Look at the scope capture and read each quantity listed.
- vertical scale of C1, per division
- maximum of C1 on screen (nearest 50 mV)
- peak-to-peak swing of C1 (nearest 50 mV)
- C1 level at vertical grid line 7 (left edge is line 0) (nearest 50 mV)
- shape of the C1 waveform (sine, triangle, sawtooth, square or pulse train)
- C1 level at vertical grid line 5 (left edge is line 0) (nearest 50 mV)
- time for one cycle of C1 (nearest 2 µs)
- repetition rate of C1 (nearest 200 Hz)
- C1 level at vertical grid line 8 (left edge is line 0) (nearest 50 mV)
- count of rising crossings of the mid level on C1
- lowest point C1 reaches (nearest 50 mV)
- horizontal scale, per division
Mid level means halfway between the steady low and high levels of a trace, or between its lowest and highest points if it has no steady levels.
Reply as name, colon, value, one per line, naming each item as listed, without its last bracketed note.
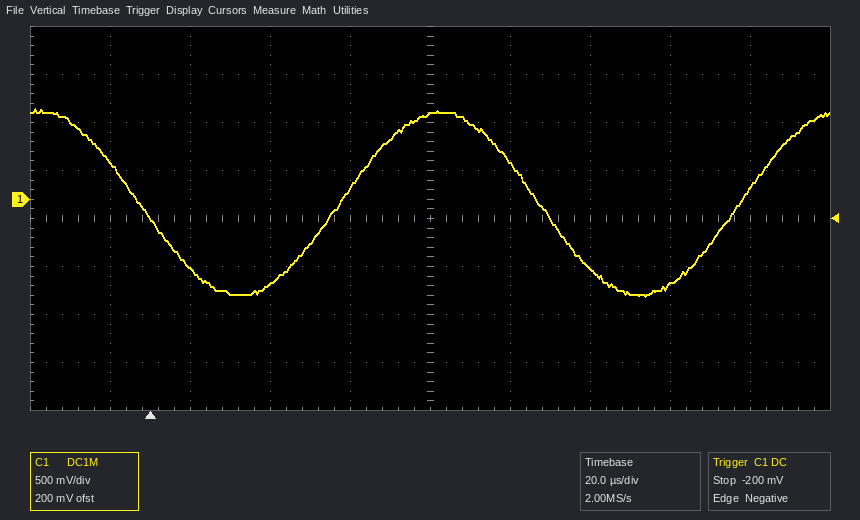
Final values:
vertical scale of C1, per division: 500 mV
maximum of C1 on screen: 950 mV
peak-to-peak swing of C1: 1.95 V
C1 level at vertical grid line 7 (left edge is line 0): -700 mV
shape of the C1 waveform: sine
C1 level at vertical grid line 5 (left edge is line 0): 900 mV
time for one cycle of C1: 100 µs
repetition rate of C1: 10.0 kHz
C1 level at vertical grid line 8 (left edge is line 0): -900 mV
count of rising crossings of the mid level on C1: 2
lowest point C1 reaches: -1.00 V
horizontal scale, per division: 20 µs
